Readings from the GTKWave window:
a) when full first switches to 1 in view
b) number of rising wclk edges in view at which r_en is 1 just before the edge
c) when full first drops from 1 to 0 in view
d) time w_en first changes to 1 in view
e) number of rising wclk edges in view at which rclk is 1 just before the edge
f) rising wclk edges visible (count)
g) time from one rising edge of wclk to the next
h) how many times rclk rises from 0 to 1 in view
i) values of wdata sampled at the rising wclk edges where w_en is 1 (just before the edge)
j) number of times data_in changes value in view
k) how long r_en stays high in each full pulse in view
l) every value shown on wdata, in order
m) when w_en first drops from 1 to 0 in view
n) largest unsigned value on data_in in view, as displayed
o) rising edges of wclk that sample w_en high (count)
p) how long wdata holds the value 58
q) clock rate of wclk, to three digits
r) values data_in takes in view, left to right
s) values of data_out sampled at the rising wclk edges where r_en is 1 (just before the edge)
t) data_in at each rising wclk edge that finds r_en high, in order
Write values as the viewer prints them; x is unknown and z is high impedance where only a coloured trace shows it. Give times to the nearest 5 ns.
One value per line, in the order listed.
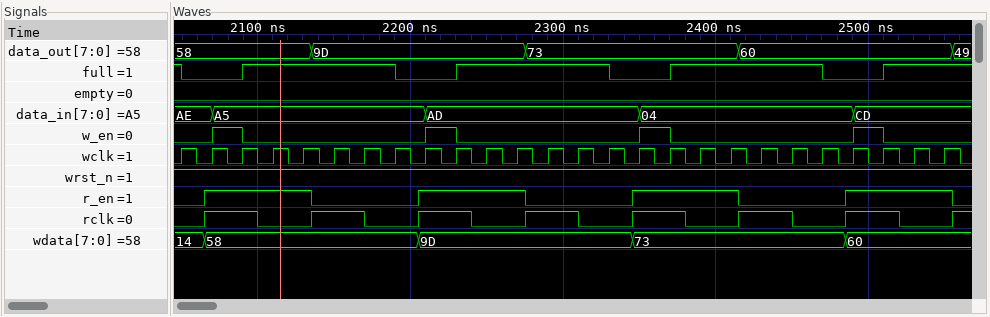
2090 ns
16
2050 ns
2070 ns
14
26
20 ns
8
58, 9D, 73, 60
4
70 ns, 70 ns, 70 ns, 70 ns
14, 58, 9D, 73, 60
2090 ns
CD
4
140 ns
50.0 MHz
AE, A5, AD, 04, CD
58, 58, 58, 58, 9D, 9D, 9D, 9D, 73, 73, 73, 73, 60, 60, 60, 60
AE, A5, A5, A5, A5, AD, AD, AD, AD, 04, 04, 04, 04, CD, CD, CD
